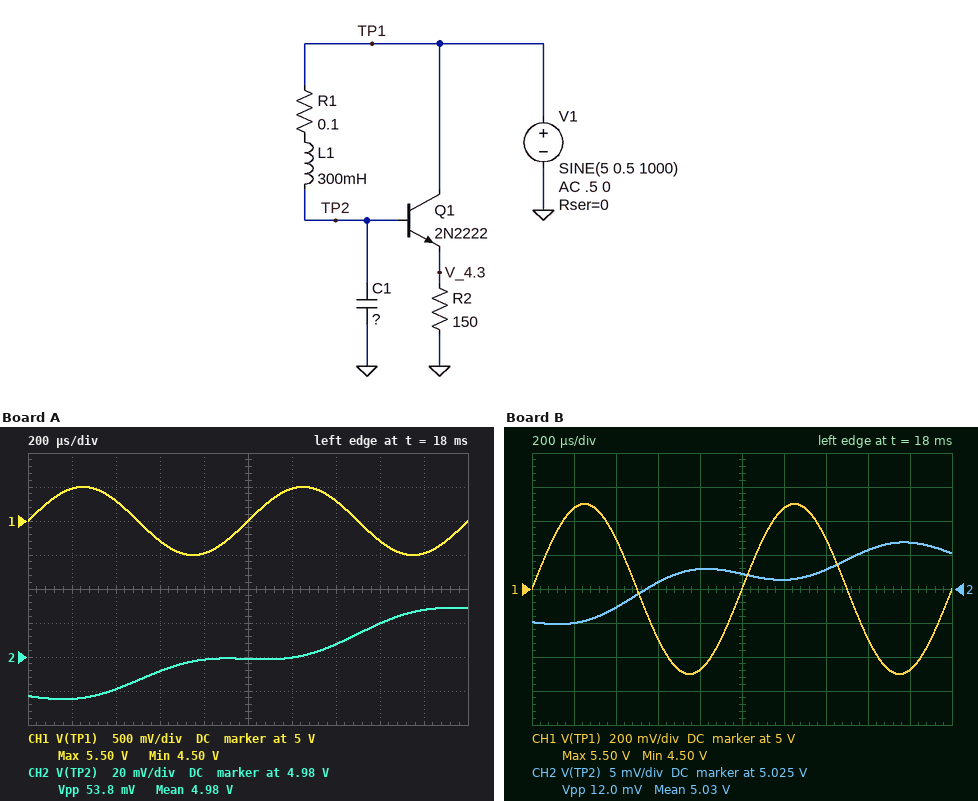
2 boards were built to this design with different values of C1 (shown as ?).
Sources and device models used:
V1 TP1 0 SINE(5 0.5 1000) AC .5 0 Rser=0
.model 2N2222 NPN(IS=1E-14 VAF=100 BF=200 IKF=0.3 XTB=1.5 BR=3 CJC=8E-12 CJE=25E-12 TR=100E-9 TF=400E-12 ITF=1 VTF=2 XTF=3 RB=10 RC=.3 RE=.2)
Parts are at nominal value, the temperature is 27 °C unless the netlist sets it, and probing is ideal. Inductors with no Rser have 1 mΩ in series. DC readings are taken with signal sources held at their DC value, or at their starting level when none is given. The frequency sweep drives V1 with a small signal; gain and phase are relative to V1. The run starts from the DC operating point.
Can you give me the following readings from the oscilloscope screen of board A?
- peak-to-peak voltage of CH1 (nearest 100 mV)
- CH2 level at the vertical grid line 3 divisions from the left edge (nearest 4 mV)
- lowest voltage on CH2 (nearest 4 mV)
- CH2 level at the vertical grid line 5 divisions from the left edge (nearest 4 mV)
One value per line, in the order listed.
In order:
1.0 V
4.972 V
4.956 V
4.980 V
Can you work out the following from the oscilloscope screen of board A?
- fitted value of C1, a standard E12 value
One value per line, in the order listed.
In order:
8.2 µF
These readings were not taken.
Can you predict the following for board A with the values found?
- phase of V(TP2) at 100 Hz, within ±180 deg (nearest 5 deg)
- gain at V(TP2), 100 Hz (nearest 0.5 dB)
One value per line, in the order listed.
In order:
-15 deg
30.5 dB
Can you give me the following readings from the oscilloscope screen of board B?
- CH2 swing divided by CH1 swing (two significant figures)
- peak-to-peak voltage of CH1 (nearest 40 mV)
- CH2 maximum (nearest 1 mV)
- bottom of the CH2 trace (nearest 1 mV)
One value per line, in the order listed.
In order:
0.012
1.00 V
5.032 V
5.020 V
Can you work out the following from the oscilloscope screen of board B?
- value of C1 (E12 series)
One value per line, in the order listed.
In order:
22 µF
